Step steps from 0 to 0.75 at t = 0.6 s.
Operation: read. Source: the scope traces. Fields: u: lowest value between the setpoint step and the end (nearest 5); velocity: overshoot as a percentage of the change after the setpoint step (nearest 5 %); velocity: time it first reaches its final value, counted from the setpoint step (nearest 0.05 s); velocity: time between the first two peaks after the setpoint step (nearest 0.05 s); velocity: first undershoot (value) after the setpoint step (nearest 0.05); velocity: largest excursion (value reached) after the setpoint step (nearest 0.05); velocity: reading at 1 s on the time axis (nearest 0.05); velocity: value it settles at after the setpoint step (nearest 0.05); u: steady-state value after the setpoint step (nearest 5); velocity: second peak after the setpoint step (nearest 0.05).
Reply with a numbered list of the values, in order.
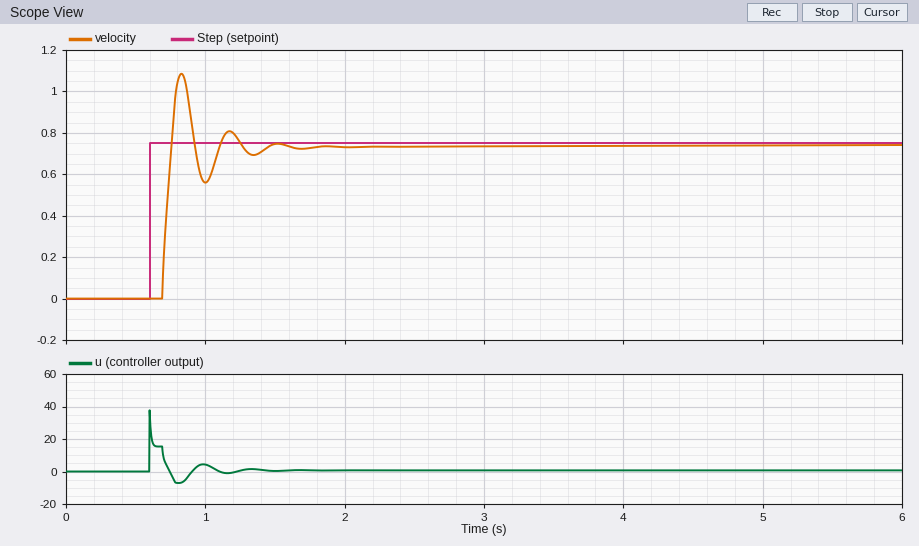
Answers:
1. -5
2. 45 %
3. 0.15 s
4. 0.35 s
5. 0.55
6. 1.10
7. 0.55
8. 0.75
9. 0
10. 0.80
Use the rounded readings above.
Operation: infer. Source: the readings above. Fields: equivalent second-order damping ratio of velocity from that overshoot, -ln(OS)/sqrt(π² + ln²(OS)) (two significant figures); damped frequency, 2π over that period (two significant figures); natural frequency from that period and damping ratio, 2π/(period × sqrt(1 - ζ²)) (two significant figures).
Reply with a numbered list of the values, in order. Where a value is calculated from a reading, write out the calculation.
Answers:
1. ln(0.45) = -0.799; 0.799 / sqrt(9.870 + 0.638) = 0.25
2. 2π / 0.35 = 18 rad/s
3. 2π / (0.35 × sqrt(1 - 0.25²)) = 19 rad/s
